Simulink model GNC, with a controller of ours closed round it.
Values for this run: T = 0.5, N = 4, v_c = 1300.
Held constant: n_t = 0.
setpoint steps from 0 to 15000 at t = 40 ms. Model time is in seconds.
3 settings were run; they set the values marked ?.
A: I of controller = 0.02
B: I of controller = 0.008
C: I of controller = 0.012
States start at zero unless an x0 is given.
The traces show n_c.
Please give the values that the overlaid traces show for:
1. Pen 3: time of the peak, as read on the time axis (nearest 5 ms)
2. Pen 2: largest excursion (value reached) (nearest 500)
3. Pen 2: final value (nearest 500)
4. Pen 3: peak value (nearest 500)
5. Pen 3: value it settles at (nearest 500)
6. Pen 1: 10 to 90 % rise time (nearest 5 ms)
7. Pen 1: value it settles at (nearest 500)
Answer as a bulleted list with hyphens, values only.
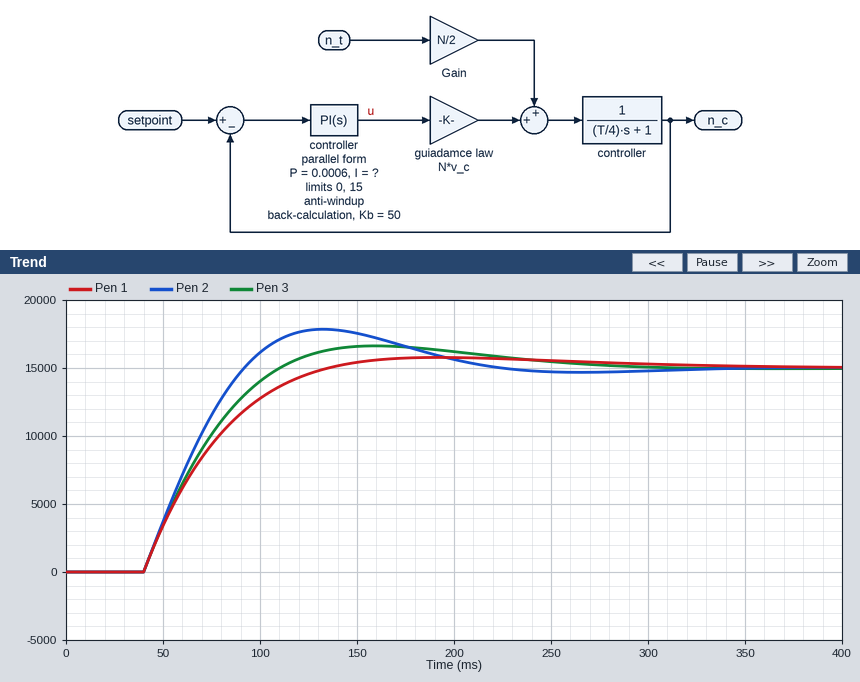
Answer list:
- 160 ms
- 18000
- 15000
- 16500
- 15000
- 65 ms
- 15000
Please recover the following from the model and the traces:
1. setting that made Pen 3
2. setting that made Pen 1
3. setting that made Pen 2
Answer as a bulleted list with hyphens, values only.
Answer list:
- C
- B
- A
